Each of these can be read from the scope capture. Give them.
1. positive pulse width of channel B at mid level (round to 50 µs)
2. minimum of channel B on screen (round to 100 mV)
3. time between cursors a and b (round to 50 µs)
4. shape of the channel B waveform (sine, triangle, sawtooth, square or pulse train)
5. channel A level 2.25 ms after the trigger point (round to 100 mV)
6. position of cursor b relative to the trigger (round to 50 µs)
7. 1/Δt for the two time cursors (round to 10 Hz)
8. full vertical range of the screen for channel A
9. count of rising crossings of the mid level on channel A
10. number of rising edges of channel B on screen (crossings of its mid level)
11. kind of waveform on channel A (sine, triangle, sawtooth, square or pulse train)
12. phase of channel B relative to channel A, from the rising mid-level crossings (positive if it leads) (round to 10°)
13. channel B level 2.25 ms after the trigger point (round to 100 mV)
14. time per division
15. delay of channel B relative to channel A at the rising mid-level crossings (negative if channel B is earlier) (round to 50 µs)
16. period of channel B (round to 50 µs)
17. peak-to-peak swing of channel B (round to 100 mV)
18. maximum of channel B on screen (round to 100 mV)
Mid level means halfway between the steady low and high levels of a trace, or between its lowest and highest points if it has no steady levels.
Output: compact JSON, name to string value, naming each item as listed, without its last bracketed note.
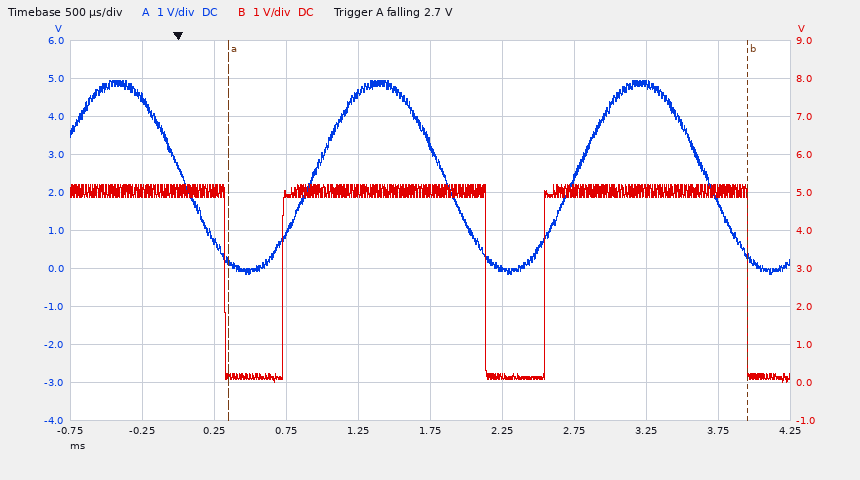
{"positive pulse width of channel B at mid level": "1.40 ms", "minimum of channel B on screen": "0.0 V", "time between cursors a and b": "3.60 ms", "shape of the channel B waveform": "pulse train", "channel A level 2.25 ms after the trigger point": "0.0 V", "position of cursor b relative to the trigger": "+3.95 ms", "1/Δt for the two time cursors": "280 Hz", "full vertical range of the screen for channel A": "10 V", "count of rising crossings of the mid level on channel A": "2", "number of rising edges of channel B on screen": "2", "kind of waveform on channel A": "sine", "phase of channel B relative to channel A, from the rising mid-level crossings (positive if it leads)": "+40°", "channel B level 2.25 ms after the trigger point": "200 mV", "time per division": "500 µs", "delay of channel B relative to channel A at the rising mid-level crossings (negative if channel B is earlier)": "-200 µs", "period of channel B": "1.80 ms", "peak-to-peak swing of channel B": "5.2 V", "maximum of channel B on screen": "5.2 V"}
